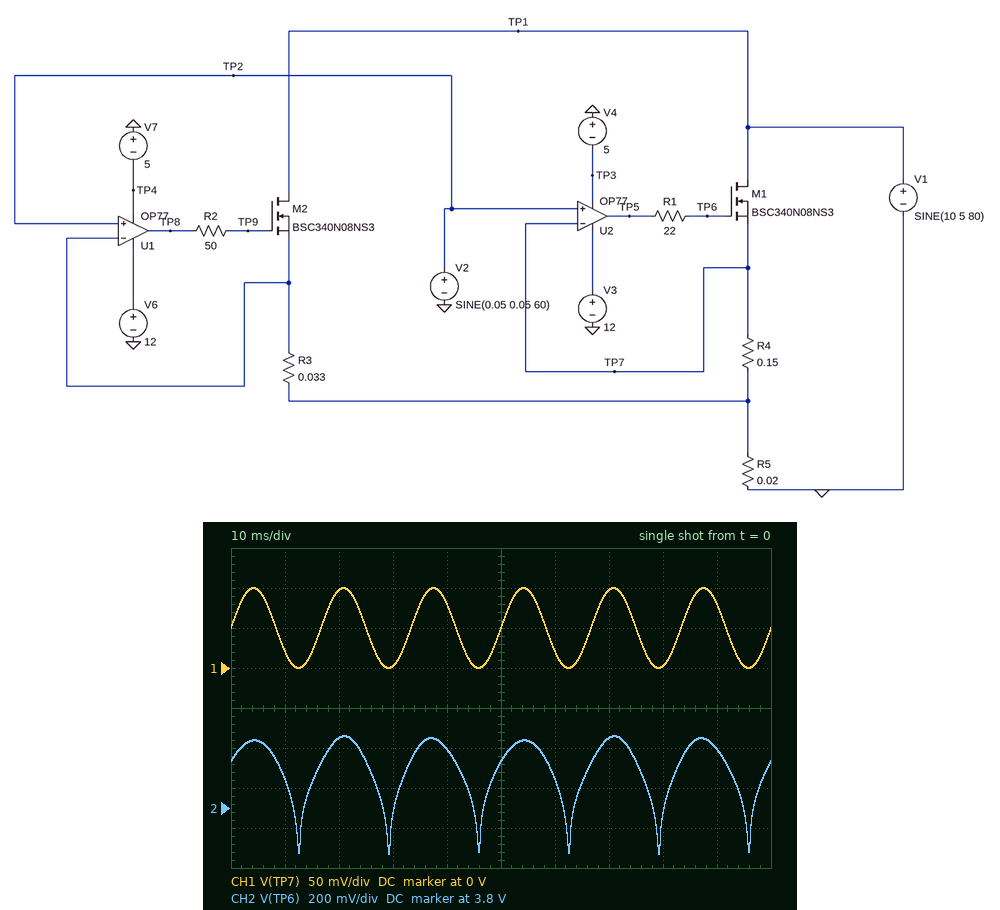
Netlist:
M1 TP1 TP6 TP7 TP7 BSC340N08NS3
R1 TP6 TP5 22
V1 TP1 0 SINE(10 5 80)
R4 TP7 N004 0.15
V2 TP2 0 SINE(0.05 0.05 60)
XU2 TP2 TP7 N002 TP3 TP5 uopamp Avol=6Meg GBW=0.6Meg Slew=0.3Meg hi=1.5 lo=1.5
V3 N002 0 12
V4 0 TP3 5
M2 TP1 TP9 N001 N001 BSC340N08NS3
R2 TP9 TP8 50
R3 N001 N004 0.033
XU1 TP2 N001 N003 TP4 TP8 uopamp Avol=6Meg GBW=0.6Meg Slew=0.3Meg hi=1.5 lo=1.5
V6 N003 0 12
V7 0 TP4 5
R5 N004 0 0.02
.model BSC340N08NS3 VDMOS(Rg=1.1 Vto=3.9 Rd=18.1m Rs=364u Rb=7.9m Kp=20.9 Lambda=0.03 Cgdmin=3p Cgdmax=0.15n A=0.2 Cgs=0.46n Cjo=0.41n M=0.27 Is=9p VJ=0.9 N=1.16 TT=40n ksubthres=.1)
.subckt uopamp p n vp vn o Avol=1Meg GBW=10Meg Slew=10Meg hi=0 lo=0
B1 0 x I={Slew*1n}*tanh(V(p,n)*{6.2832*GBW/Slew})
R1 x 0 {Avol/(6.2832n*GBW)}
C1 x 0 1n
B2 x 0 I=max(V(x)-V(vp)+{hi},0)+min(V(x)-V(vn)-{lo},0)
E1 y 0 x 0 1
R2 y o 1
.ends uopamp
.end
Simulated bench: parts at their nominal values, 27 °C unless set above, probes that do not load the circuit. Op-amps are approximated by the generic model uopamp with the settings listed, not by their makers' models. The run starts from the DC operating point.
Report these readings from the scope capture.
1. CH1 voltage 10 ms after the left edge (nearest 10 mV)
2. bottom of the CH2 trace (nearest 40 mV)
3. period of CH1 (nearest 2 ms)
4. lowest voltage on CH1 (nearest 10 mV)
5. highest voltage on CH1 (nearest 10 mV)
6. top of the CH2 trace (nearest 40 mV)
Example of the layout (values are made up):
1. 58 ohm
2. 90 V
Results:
1. 20 mV
2. 3.56 V
3. 16 ms
4. 0 V
5. 100 mV
6. 4.16 V
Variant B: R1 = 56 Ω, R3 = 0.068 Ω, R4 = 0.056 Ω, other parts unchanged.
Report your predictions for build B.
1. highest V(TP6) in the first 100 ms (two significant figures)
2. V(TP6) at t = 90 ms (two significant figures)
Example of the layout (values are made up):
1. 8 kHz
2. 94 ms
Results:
1. 4.3 V
2. 4.2 V
